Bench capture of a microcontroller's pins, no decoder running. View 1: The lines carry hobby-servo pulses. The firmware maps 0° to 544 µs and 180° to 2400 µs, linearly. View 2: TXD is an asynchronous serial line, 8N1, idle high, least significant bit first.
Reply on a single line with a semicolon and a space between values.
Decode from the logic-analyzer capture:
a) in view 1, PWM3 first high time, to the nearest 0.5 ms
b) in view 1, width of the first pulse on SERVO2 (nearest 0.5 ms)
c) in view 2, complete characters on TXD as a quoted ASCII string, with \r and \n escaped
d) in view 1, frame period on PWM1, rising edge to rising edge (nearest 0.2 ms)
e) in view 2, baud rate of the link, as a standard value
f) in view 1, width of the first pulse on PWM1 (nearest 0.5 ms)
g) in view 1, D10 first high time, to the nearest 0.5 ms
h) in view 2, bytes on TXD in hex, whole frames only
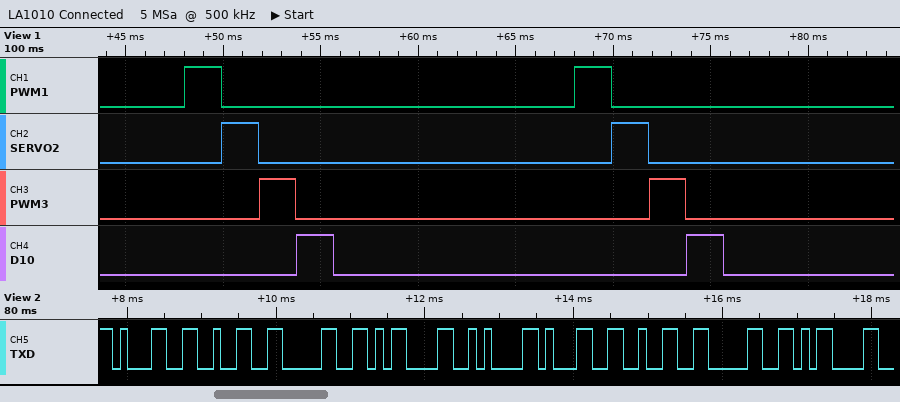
2.0 ms; 2.0 ms; "120\r\n120\r"; 20.0 ms; 9600 baud; 2.0 ms; 2.0 ms; 0x31 0x32 0x30 0x0D 0x0A 0x31 0x32 0x30 0x0D
